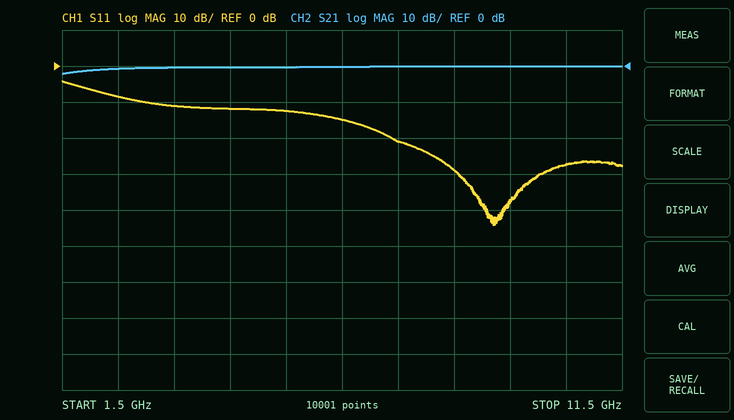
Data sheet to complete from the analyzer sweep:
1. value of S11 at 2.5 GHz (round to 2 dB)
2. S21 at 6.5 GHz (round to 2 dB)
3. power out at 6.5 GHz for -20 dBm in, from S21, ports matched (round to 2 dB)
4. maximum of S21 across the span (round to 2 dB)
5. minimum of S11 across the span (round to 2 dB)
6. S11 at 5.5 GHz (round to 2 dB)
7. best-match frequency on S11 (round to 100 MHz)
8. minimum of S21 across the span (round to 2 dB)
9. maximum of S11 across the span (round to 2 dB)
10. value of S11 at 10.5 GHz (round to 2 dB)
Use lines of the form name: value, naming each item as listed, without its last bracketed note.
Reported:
value of S11 at 2.5 GHz: -8 dB
S21 at 6.5 GHz: 0 dB
power out at 6.5 GHz for -20 dBm in, from S21, ports matched: -20 dBm
maximum of S21 across the span: 0 dB
minimum of S11 across the span: -44 dB
S11 at 5.5 GHz: -12 dB
best-match frequency on S11: 9.2 GHz
minimum of S21 across the span: -2 dB
maximum of S11 across the span: -4 dB
value of S11 at 10.5 GHz: -28 dB
